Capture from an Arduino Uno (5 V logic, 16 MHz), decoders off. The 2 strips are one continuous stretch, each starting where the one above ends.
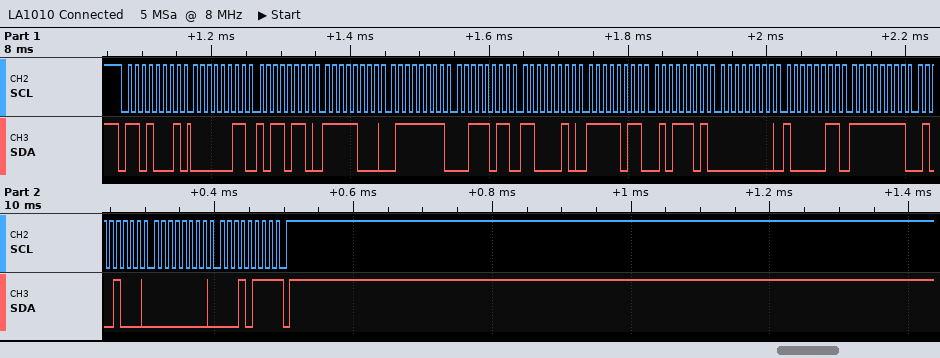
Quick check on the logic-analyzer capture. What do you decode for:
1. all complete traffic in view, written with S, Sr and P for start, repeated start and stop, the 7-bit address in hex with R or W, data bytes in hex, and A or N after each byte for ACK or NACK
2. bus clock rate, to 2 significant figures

S 68R A 03 A B6 A F8 A 7F A 3B A C2 A FB A 5D A 00 A 83 A FF A 48 A 00 A 17 N P
100 kHz
